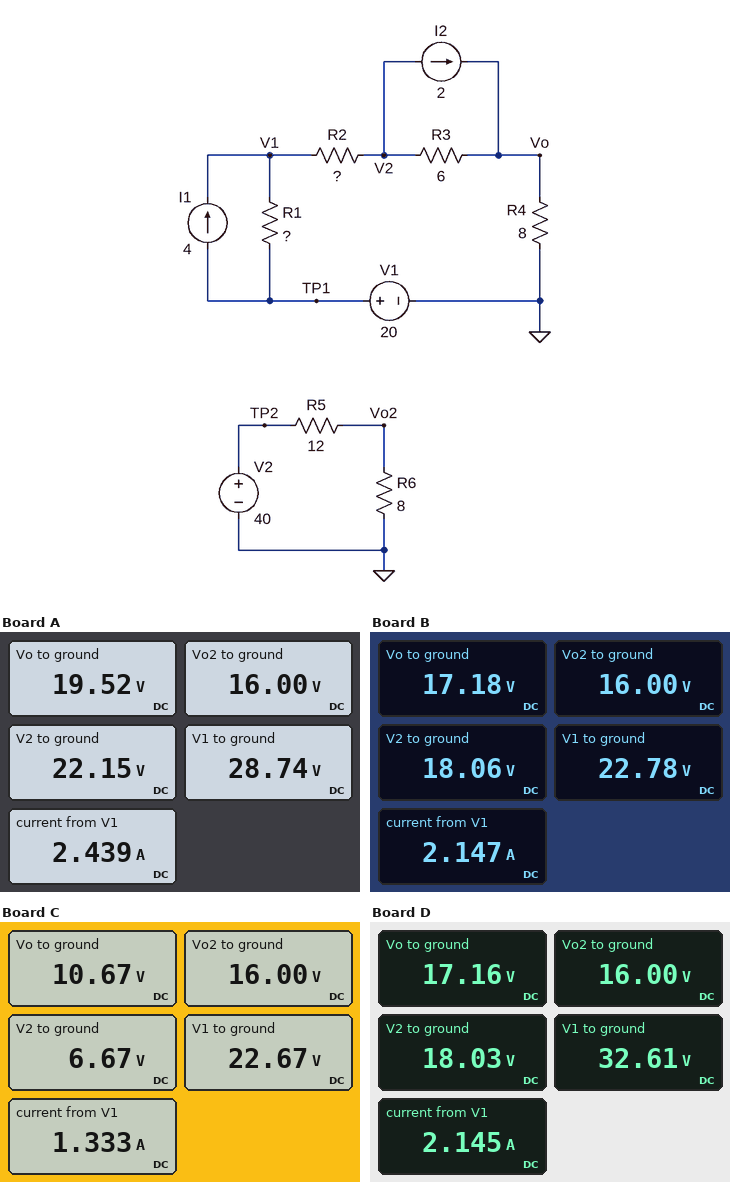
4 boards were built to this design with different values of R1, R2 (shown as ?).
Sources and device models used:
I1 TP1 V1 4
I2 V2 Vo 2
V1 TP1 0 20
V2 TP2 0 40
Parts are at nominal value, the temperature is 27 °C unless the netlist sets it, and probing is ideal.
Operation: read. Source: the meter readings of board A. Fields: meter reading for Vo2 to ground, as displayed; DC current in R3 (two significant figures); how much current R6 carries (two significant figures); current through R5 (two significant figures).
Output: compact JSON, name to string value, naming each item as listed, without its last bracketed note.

{"meter reading for Vo2 to ground, as displayed": "16.00 V", "DC current in R3": "440 mA", "how much current R6 carries": "2.0 A", "current through R5": "2.0 A"}
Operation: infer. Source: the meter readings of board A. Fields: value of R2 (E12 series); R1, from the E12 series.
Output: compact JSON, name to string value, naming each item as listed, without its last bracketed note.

{"value of R2": "2.7 Ω", "R1, from the E12 series": "5.6 Ω"}
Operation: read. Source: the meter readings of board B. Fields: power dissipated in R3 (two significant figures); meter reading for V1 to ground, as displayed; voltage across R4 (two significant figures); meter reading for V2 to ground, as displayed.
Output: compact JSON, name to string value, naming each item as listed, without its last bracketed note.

{"power dissipated in R3": "130 mW", "meter reading for V1 to ground, as displayed": "22.78 V", "voltage across R4": "17 V", "meter reading for V2 to ground, as displayed": "18.06 V"}
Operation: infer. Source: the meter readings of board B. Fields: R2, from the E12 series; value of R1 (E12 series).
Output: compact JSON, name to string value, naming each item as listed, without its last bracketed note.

{"R2, from the E12 series": "2.2 Ω", "value of R1": "1.5 Ω"}
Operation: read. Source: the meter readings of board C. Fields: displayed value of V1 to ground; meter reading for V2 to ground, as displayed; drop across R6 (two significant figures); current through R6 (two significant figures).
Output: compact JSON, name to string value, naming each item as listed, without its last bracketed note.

{"displayed value of V1 to ground": "22.67 V", "meter reading for V2 to ground, as displayed": "6.67 V", "drop across R6": "16 V", "current through R6": "2.0 A"}
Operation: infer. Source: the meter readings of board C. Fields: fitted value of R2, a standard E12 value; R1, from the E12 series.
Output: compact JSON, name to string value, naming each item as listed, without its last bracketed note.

{"fitted value of R2, a standard E12 value": "12 Ω", "R1, from the E12 series": "1 Ω"}
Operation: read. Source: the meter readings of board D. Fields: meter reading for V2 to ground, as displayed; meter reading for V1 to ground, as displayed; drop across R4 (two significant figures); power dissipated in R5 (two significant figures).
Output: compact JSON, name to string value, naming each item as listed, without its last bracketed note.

{"meter reading for V2 to ground, as displayed": "18.03 V", "meter reading for V1 to ground, as displayed": "32.61 V", "drop across R4": "17 V", "power dissipated in R5": "48 W"}
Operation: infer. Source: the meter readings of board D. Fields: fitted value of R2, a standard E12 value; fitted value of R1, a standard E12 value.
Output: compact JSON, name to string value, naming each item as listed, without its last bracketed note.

{"fitted value of R2, a standard E12 value": "6.8 Ω", "fitted value of R1, a standard E12 value": "6.8 Ω"}
